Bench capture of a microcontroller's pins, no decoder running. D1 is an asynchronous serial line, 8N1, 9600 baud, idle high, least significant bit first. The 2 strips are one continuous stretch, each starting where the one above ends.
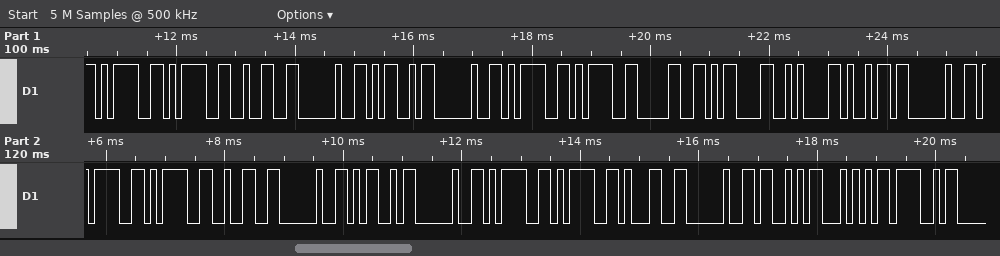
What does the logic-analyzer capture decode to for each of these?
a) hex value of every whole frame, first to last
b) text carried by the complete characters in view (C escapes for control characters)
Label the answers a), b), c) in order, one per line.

a) 3D 3D 32 20 4D 20 3D 3D 30 0D 0A 69 20 3D 3D 32 20 4D 20 3D 3D 31 20 53 54 4F
b) "==2 M ==0\r\ni ==2 M ==1 STO"
